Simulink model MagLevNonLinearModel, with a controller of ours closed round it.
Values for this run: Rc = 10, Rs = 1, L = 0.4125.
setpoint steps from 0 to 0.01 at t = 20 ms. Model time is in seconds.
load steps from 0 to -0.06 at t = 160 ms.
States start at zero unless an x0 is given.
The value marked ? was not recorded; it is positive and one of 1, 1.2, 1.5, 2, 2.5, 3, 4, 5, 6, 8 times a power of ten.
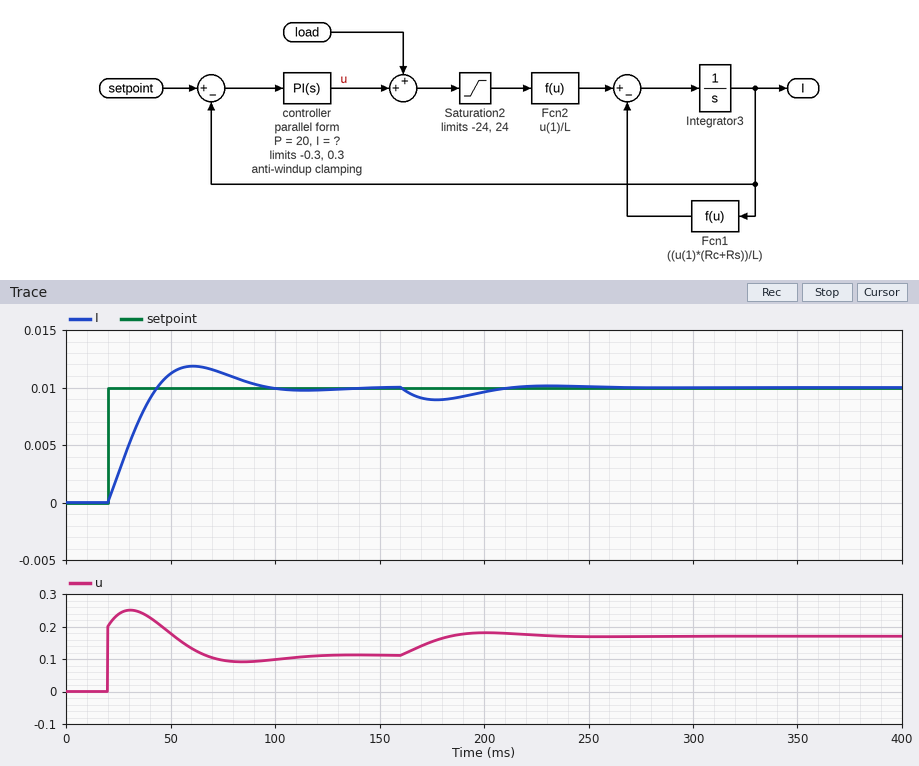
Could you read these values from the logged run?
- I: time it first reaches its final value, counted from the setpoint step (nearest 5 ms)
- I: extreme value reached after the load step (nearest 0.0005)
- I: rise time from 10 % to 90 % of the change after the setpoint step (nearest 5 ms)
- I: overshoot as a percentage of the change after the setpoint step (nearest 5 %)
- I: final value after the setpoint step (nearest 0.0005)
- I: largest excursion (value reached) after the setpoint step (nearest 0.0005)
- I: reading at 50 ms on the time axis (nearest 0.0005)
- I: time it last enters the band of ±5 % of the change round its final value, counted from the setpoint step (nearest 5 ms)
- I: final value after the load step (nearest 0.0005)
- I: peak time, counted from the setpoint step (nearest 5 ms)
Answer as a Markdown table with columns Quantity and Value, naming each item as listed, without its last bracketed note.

| Quantity | Value |
|---|---|
| I: time it first reaches its final value, counted from the setpoint step | 25 ms |
| I: extreme value reached after the load step | 0.0090 |
| I: rise time from 10 % to 90 % of the change after the setpoint step | 20 ms |
| I: overshoot as a percentage of the change after the setpoint step | 20 % |
| I: final value after the setpoint step | 0.0100 |
| I: largest excursion (value reached) after the setpoint step | 0.0120 |
| I: reading at 50 ms on the time axis | 0.0110 |
| I: time it last enters the band of ±5 % of the change round its final value, counted from the setpoint step | 65 ms |
| I: final value after the load step | 0.0100 |
| I: peak time, counted from the setpoint step | 40 ms |
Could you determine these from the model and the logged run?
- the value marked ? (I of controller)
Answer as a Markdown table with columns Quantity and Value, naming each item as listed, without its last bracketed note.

| Quantity | Value |
|---|---|
| the value marked ? | 2000 |
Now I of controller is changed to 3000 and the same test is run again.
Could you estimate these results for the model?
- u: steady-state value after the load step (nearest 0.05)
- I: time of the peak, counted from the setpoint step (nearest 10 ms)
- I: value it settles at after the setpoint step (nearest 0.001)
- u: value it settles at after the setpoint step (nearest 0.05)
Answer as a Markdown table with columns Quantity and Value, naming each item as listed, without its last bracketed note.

| Quantity | Value |
|---|---|
| u: steady-state value after the load step | 0.15 |
| I: time of the peak, counted from the setpoint step | 30 ms |
| I: value it settles at after the setpoint step | 0.010 |
| u: value it settles at after the setpoint step | 0.10 |
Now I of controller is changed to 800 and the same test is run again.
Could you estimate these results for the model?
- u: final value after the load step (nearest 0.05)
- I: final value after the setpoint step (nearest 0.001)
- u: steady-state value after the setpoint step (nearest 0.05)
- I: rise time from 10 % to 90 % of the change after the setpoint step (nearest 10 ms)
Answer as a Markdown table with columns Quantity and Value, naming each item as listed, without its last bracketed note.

| Quantity | Value |
|---|---|
| u: final value after the load step | 0.15 |
| I: final value after the setpoint step | 0.010 |
| u: steady-state value after the setpoint step | 0.10 |
| I: rise time from 10 % to 90 % of the change after the setpoint step | 30 ms |
